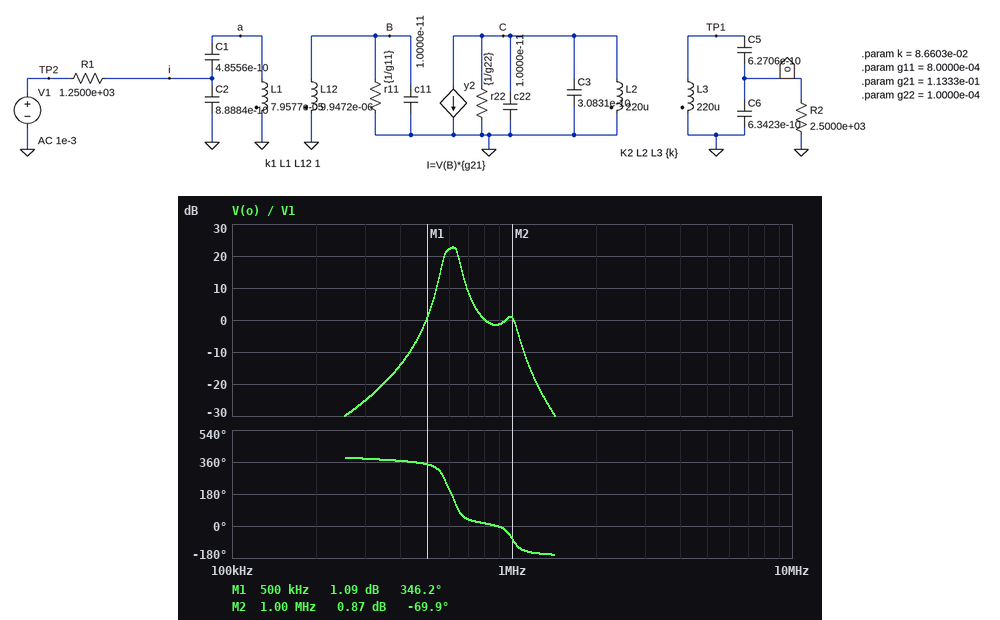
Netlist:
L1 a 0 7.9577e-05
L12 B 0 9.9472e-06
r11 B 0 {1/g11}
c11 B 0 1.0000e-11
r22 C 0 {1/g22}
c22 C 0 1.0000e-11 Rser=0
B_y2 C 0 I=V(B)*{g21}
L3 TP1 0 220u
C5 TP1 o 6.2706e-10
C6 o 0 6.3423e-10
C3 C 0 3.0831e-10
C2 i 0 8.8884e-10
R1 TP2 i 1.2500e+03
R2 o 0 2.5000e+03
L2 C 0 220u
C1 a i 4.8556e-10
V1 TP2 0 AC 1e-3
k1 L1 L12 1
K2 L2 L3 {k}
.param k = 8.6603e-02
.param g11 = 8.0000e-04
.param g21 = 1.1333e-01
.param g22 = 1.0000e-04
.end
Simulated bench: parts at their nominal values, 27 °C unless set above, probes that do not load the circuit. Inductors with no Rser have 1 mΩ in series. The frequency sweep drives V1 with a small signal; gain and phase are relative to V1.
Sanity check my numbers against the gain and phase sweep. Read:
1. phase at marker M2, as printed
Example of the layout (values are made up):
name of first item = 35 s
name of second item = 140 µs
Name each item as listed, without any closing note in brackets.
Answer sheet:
phase at marker M2, as printed = -69.9 deg
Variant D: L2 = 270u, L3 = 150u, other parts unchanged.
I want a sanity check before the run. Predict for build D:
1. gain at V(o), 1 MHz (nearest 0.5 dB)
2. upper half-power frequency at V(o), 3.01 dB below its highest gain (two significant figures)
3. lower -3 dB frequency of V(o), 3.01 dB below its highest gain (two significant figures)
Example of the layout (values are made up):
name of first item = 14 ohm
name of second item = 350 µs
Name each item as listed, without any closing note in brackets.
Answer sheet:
gain at V(o), 1 MHz = 3.5 dB
upper half-power frequency at V(o), 3.01 dB below its highest gain = 760 kHz
lower -3 dB frequency of V(o), 3.01 dB below its highest gain = 710 kHz
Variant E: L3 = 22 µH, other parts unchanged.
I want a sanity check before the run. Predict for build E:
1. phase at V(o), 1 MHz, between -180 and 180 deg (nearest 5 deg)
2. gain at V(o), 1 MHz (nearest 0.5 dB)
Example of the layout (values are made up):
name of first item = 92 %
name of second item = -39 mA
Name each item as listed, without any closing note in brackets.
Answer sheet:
phase at V(o), 1 MHz, between -180 and 180 deg = 105 deg
gain at V(o), 1 MHz = -1.5 dB
